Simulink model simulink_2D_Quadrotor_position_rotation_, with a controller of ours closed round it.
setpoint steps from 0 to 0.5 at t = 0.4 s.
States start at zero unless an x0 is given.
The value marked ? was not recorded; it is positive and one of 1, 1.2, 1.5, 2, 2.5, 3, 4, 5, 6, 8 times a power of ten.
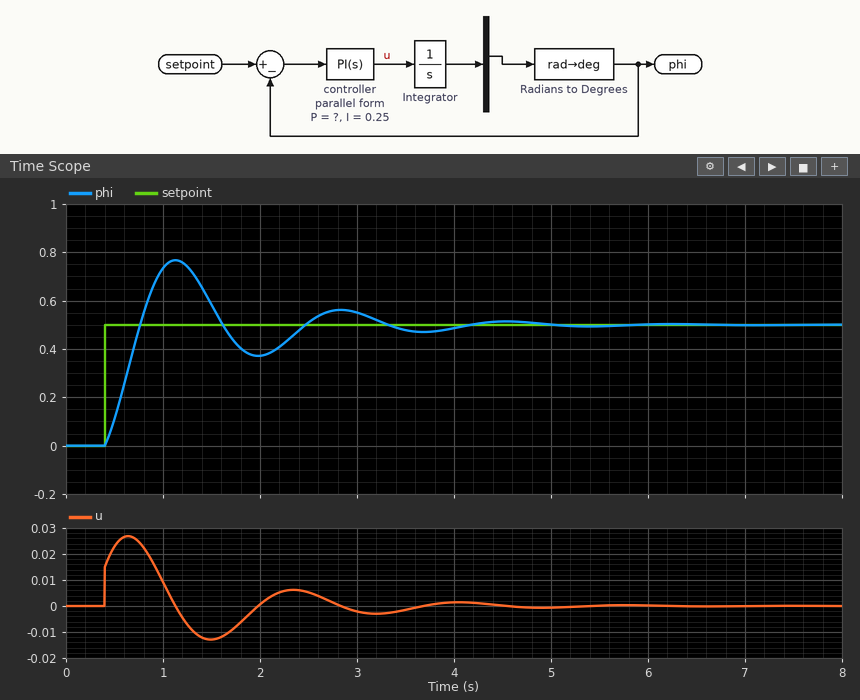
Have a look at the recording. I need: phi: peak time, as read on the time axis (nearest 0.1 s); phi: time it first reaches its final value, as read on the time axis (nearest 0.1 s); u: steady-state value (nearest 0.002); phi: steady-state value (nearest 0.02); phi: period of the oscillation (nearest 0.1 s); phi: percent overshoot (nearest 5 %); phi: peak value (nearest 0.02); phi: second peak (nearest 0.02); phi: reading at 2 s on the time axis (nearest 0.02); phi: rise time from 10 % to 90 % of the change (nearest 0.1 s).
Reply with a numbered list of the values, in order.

1. 1.1 s
2. 0.8 s
3. 0.000
4. 0.50
5. 1.7 s
6. 55 %
7. 0.76
8. 0.56
9. 0.38
10. 0.3 s
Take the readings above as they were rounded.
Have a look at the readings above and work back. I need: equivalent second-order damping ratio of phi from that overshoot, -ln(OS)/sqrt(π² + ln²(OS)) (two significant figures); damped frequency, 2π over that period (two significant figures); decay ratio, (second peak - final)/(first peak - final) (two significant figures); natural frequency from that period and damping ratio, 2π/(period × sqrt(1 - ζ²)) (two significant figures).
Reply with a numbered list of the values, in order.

1. 0.19
2. 3.7 rad/s
3. 0.23
4. 3.8 rad/s
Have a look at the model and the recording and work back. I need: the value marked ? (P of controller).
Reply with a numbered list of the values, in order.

1. 0.03
